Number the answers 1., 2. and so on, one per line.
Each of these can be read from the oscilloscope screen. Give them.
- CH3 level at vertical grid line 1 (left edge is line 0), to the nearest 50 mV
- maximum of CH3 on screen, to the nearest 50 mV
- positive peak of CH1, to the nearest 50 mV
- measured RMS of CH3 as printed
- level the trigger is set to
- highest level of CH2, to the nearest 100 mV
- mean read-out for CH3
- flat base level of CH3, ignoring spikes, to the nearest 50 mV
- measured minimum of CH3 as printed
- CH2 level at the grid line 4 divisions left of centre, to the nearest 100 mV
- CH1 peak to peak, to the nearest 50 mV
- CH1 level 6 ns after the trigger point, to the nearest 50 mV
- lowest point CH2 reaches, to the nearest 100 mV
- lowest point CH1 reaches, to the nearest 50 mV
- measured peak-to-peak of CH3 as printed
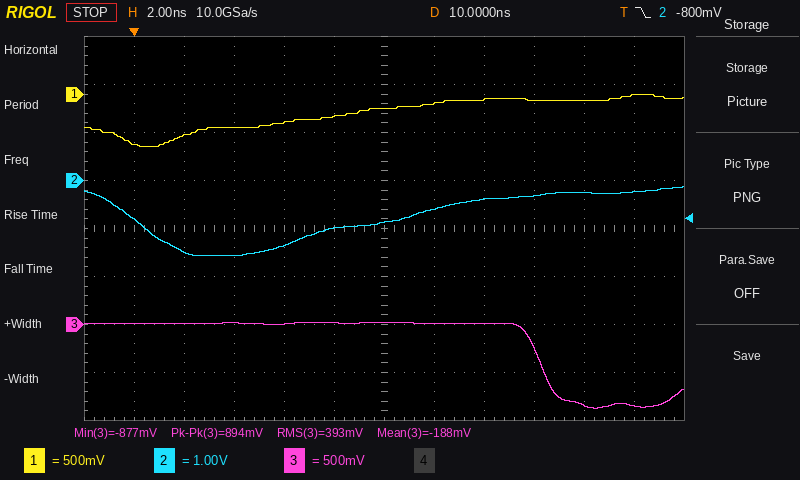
1. 0 mV
2. 0 mV
3. 0 mV
4. 393 mV
5. -800 mV
6. -100 mV
7. -188 mV
8. -850 mV
9. -877 mV
10. -1.5 V
11. 550 mV
12. -300 mV
13. -1.6 V
14. -550 mV
15. 894 mV
